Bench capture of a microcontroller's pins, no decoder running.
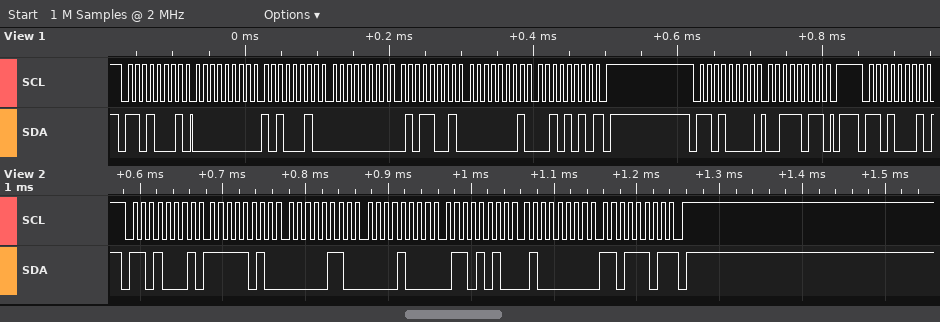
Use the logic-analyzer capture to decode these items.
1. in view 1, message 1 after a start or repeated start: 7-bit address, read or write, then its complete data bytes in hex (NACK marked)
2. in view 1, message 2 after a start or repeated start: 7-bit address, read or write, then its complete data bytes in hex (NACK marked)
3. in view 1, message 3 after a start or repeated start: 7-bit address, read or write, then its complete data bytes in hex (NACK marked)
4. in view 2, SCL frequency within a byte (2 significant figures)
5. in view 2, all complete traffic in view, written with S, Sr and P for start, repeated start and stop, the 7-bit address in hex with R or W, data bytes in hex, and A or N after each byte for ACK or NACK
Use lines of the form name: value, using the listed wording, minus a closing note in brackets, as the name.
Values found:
in view 1, message 1 after a start or repeated start: 7-bit address, read or write, then its complete data bytes in hex: 0x68 read: 00 A2 00 59 01 2A NACK
in view 1, message 2 after a start or repeated start: 7-bit address, read or write, then its complete data bytes in hex: 0x68 write: 3B
in view 1, message 3 after a start or repeated start: 7-bit address, read or write, then its complete data bytes in hex: 0x68 read
in view 2, SCL frequency within a byte: 100 kHz
in view 2, all complete traffic in view, written with S, Sr and P for start, repeated start and stop, the 7-bit address in hex with R or W, data bytes in hex, and A or N after each byte for ACK or NACK: S 68R A FA A 06 A 08 A 6A A 40 A DD N P
